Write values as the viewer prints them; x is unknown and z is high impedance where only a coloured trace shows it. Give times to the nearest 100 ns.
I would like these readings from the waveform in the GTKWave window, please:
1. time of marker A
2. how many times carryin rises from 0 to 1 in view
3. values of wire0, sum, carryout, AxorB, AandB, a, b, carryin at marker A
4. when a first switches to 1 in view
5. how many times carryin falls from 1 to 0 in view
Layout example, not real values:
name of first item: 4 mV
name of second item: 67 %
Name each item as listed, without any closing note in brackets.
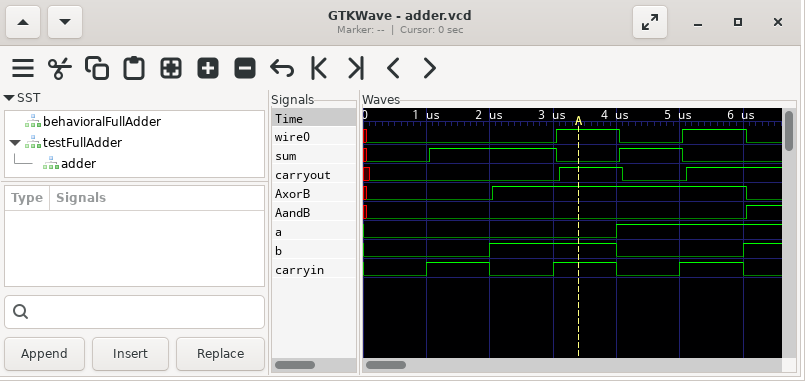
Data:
time of marker A: 3400 ns
how many times carryin rises from 0 to 1 in view: 3
values of wire0, sum, carryout, AxorB, AandB, a, b, carryin at marker A: wire0=1, sum=0, carryout=1, AxorB=1, AandB=0, a=0, b=1, carryin=1
when a first switches to 1 in view: 4000 ns
how many times carryin falls from 1 to 0 in view: 3
